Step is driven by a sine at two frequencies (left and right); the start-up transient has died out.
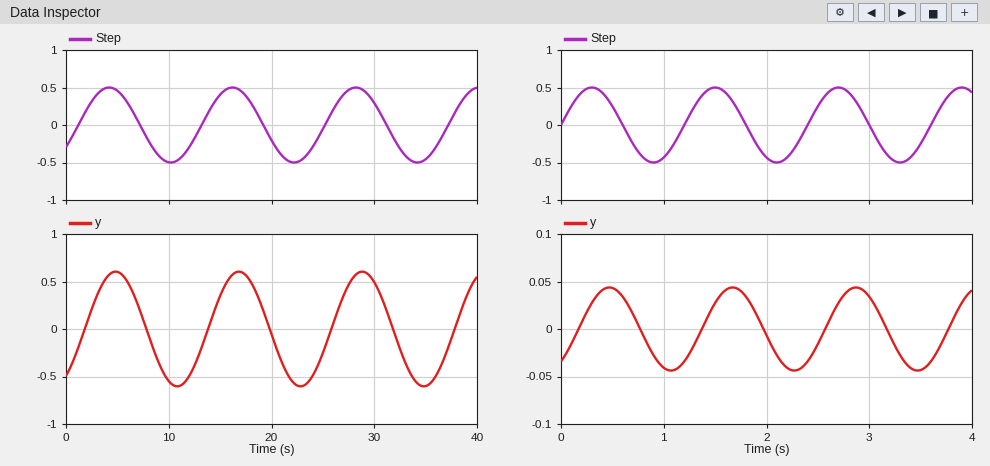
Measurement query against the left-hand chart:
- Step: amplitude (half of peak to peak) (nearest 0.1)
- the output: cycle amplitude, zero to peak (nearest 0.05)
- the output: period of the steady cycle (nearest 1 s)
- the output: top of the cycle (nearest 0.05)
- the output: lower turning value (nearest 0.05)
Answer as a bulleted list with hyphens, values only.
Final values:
- 0.5
- 0.60
- 12 s
- 0.60
- -0.60
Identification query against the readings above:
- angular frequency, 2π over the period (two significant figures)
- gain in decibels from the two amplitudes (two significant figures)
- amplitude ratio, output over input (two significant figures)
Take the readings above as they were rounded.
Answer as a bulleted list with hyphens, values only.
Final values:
- 0.52 rad/s
- 1.6 dB
- 1.2
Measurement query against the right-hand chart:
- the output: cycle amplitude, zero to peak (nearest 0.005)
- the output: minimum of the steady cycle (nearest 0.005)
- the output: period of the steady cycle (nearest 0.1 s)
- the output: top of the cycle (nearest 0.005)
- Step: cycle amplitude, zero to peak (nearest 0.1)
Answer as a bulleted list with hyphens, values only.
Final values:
- 0.045
- -0.045
- 1.2 s
- 0.045
- 0.5
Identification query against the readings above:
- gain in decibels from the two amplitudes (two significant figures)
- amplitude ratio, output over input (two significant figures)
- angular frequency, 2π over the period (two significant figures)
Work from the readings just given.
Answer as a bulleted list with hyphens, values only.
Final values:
- -21 dB
- 0.090
- 5.2 rad/s
